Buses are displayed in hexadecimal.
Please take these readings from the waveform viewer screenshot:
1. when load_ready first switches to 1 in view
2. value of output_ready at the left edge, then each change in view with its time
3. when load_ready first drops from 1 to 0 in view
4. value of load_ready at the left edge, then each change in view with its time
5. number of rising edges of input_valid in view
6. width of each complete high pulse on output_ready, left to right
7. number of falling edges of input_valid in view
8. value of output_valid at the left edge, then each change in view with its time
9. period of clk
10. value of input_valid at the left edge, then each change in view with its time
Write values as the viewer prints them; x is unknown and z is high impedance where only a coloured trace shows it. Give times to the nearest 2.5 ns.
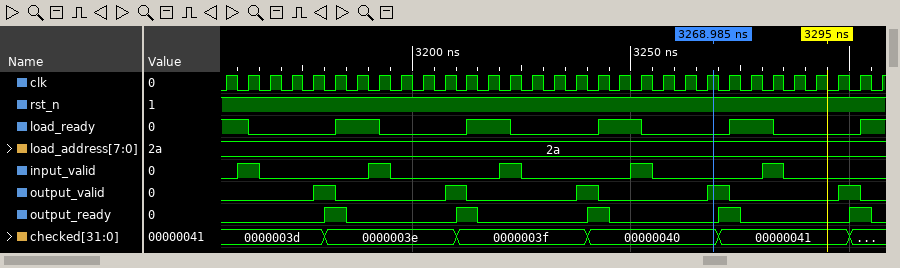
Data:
3182.5 ns
0, 1 at 3180 ns, 0 at 3185 ns, 1 at 3210 ns, 0 at 3215 ns, 1 at 3240 ns, 0 at 3245 ns, 1 at 3270 ns, 0 at 3275 ns, 1 at 3300 ns, 0 at 3305 ns
3162.5 ns
1, 0 at 3162.5 ns, 1 at 3182.5 ns, 0 at 3192.5 ns, 1 at 3212.5 ns, 0 at 3222.5 ns, 1 at 3242.5 ns, 0 at 3252.5 ns, 1 at 3272.5 ns, 0 at 3282.5 ns, 1 at 3302.5 ns
5
5 ns, 5 ns, 5 ns, 5 ns, 5 ns
5
0, 1 at 3177.5 ns, 0 at 3182.5 ns, 1 at 3207.5 ns, 0 at 3212.5 ns, 1 at 3237.5 ns, 0 at 3242.5 ns, 1 at 3267.5 ns, 0 at 3272.5 ns, 1 at 3297.5 ns, 0 at 3302.5 ns
5 ns
0, 1 at 3160 ns, 0 at 3165 ns, 1 at 3190 ns, 0 at 3195 ns, 1 at 3220 ns, 0 at 3225 ns, 1 at 3250 ns, 0 at 3255 ns, 1 at 3280 ns, 0 at 3285 ns
